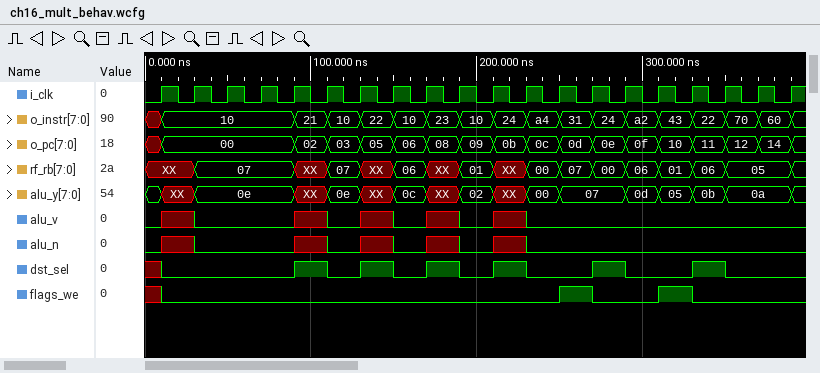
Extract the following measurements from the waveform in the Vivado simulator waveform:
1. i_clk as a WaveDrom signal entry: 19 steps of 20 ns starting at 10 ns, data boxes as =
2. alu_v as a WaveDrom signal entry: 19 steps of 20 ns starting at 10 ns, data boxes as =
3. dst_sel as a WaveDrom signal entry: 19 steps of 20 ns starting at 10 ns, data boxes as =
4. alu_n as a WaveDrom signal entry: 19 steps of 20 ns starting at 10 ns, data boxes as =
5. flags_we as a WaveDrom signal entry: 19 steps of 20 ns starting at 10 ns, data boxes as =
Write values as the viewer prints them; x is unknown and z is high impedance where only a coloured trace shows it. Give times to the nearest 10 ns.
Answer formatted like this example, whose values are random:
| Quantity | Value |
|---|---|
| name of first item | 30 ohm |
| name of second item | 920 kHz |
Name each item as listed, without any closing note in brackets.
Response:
| Quantity | Value |
|---|---|
| i_clk as a WaveDrom signal entry: 19 steps of 20 ns starting at 10 ns, data boxes as = | {name: 'i_clk', wave: 'p..................'} |
| alu_v as a WaveDrom signal entry: 19 steps of 20 ns starting at 10 ns, data boxes as = | {name: 'alu_v', wave: 'x0..x0x0x0x0.......'} |
| dst_sel as a WaveDrom signal entry: 19 steps of 20 ns starting at 10 ns, data boxes as = | {name: 'dst_sel', wave: '0...10101010.10.10.'} |
| alu_n as a WaveDrom signal entry: 19 steps of 20 ns starting at 10 ns, data boxes as = | {name: 'alu_n', wave: 'x0..x0x0x0x0.......'} |
| flags_we as a WaveDrom signal entry: 19 steps of 20 ns starting at 10 ns, data boxes as = | {name: 'flags_we', wave: '0...........10.10..'} |
